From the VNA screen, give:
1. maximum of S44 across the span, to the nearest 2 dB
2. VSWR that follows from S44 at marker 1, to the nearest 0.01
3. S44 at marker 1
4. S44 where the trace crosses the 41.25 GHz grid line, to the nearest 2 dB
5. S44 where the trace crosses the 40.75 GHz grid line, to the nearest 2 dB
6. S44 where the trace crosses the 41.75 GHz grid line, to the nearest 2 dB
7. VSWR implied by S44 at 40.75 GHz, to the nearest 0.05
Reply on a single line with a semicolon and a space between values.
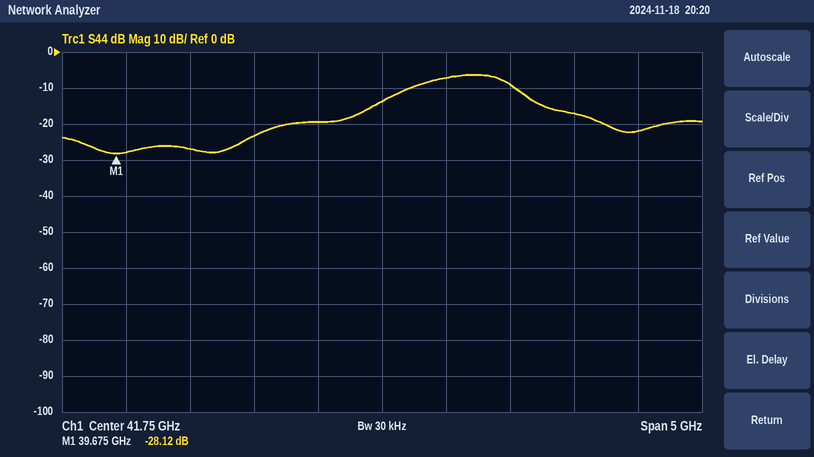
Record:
-6 dB; 1.08; -28.12 dB; -20 dB; -24 dB; -14 dB; 1.15
